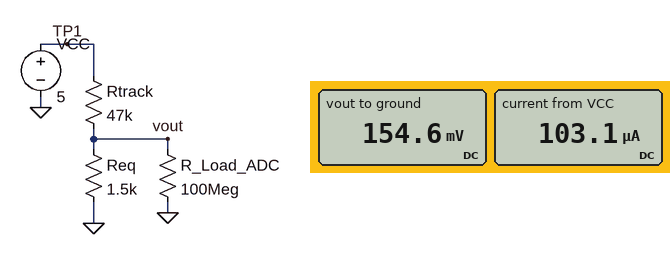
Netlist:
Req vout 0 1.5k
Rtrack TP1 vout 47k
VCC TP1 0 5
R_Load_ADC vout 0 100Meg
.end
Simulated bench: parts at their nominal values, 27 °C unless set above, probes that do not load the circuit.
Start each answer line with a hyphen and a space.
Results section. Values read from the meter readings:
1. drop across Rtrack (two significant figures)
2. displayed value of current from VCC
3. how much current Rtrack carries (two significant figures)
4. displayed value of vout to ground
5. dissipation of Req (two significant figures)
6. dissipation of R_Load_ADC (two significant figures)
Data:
- 4.8 V
- 103.1 µA
- 100 µA
- 154.6 mV
- 16 µW
- 240 pW
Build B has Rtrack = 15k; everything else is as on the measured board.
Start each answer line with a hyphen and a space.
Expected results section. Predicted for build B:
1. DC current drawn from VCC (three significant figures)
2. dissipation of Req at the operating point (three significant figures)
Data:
- 303 µA
- 138 µW
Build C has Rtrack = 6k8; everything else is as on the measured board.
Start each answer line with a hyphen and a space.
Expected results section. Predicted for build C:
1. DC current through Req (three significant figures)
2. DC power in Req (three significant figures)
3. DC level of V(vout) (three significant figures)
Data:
- 602 µA
- 544 µW
- 904 mV
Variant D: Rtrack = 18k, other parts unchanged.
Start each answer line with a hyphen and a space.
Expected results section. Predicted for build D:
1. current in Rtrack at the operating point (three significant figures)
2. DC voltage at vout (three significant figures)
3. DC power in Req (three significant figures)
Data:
- 256 µA
- 385 mV
- 98.6 µW
